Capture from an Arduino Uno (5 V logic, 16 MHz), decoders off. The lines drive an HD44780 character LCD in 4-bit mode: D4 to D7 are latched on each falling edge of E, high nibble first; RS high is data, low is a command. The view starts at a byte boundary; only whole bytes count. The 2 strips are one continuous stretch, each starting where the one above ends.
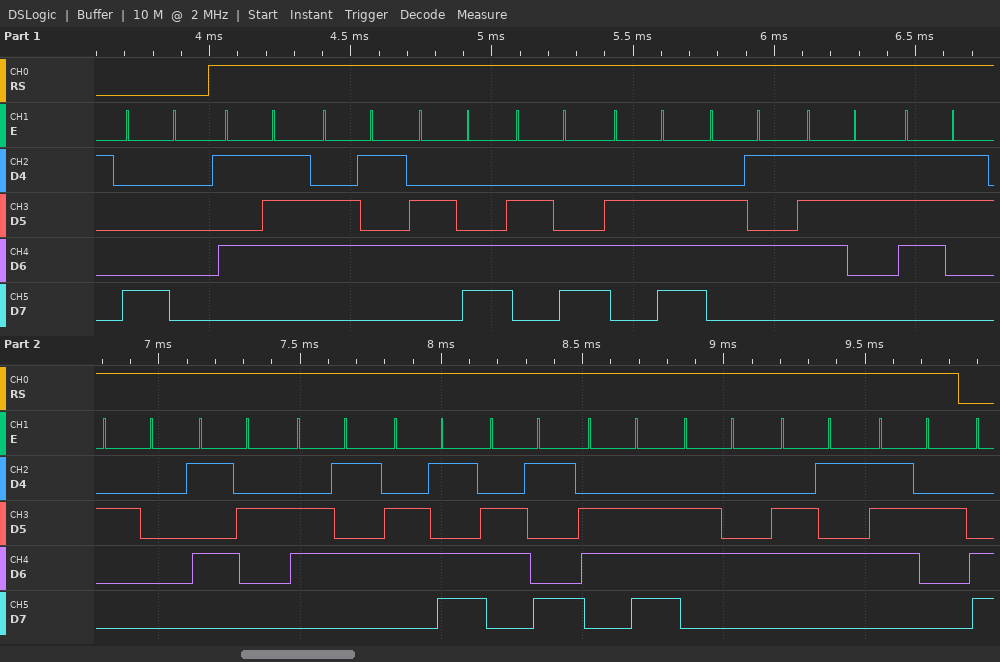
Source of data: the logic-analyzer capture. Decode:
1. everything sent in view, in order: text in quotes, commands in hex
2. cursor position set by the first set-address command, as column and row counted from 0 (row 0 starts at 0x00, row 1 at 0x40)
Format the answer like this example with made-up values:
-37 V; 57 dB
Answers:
0x80 "Wellness Reminder"; column 0, row 0
